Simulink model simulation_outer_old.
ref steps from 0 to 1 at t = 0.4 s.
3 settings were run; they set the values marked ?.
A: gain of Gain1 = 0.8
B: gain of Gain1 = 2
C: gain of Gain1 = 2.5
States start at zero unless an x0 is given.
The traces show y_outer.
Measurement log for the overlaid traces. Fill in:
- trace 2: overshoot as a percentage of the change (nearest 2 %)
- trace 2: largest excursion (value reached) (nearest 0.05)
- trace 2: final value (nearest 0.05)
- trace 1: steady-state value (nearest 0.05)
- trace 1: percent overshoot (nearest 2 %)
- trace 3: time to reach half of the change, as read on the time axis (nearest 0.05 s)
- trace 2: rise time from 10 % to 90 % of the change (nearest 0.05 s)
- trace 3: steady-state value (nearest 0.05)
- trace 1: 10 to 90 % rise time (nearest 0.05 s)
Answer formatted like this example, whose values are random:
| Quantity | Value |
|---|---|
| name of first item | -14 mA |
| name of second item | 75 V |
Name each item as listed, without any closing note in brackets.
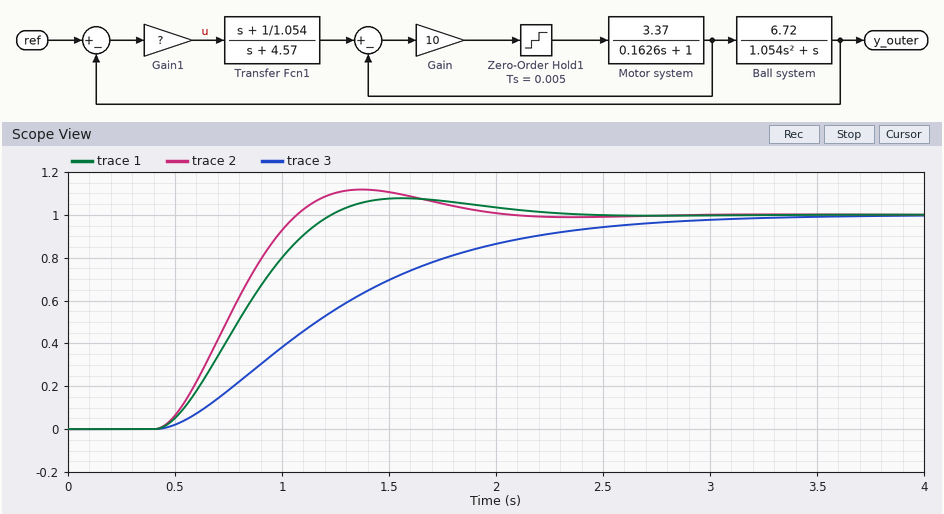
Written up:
| Quantity | Value |
|---|---|
| trace 2: overshoot as a percentage of the change | 12 % |
| trace 2: largest excursion (value reached) | 1.10 |
| trace 2: final value | 1.00 |
| trace 1: steady-state value | 1.00 |
| trace 1: percent overshoot | 8 % |
| trace 3: time to reach half of the change, as read on the time axis | 1.15 s |
| trace 2: rise time from 10 % to 90 % of the change | 0.45 s |
| trace 3: steady-state value | 1.00 |
| trace 1: 10 to 90 % rise time | 0.55 s |
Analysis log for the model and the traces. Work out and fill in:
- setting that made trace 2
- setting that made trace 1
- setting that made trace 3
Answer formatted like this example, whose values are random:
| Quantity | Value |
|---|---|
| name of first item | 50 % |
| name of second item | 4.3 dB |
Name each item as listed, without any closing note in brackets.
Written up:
| Quantity | Value |
|---|---|
| setting that made trace 2 | C |
| setting that made trace 1 | B |
| setting that made trace 3 | A |
